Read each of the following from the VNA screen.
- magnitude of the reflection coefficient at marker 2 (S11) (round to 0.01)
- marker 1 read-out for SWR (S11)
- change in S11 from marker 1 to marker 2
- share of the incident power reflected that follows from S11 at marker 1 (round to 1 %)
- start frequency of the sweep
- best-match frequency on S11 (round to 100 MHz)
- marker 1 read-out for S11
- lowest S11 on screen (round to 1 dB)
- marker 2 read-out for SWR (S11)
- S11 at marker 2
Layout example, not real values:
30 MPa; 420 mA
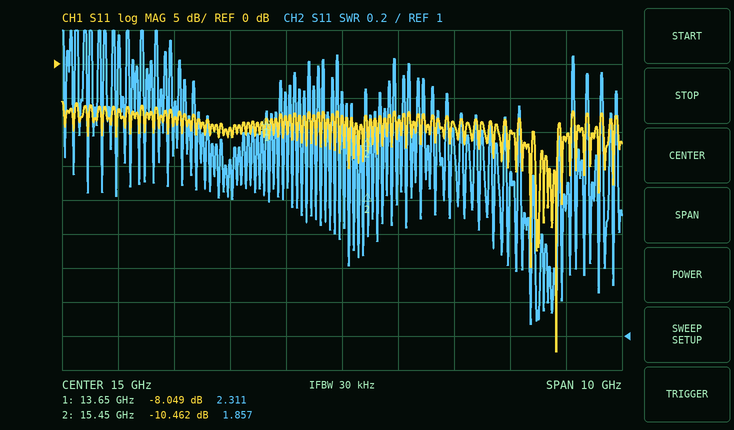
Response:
0.30; 2.311; -2.413 dB; 16 %; 10 GHz; 18.8 GHz; -8.049 dB; -42 dB; 1.857; -10.462 dB
